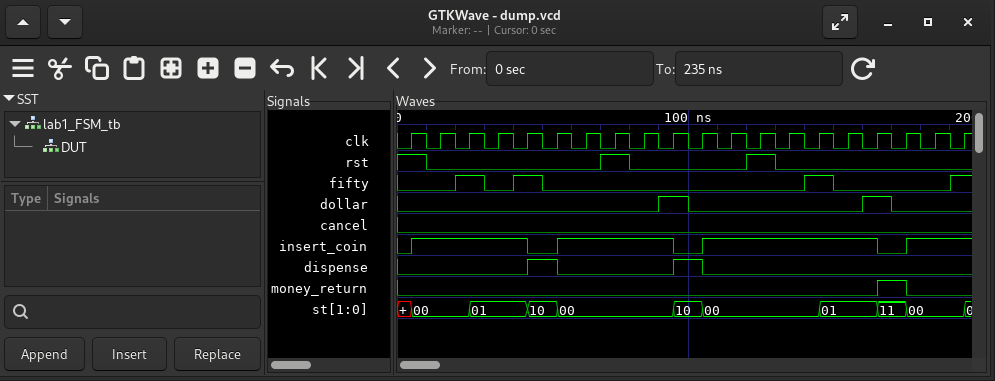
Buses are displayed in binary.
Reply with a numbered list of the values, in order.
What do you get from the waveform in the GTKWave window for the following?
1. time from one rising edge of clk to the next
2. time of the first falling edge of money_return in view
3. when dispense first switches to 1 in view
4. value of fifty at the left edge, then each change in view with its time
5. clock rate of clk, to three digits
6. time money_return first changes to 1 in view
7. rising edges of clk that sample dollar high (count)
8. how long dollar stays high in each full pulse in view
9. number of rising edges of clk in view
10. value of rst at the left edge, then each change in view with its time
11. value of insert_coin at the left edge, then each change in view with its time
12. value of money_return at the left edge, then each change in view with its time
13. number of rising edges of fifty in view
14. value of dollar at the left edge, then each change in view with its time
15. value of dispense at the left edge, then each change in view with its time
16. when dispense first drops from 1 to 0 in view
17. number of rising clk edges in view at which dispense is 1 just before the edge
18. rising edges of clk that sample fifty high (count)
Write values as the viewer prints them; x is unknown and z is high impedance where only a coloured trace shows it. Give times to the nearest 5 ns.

1. 10 ns
2. 175 ns
3. 45 ns
4. 0, 1 at 20 ns, 0 at 30 ns, 1 at 40 ns, 0 at 50 ns, 1 at 140 ns, 0 at 150 ns, 1 at 190 ns
5. 100 MHz
6. 165 ns
7. 2
8. 10 ns, 10 ns
9. 20
10. 1, 0 at 10 ns, 1 at 70 ns, 0 at 80 ns, 1 at 120 ns, 0 at 130 ns
11. 0, 1 at 5 ns, 0 at 45 ns, 1 at 55 ns, 0 at 95 ns, 1 at 105 ns, 0 at 165 ns, 1 at 175 ns
12. 0, 1 at 165 ns, 0 at 175 ns
13. 4
14. 0, 1 at 90 ns, 0 at 100 ns, 1 at 160 ns, 0 at 170 ns
15. 0, 1 at 45 ns, 0 at 55 ns, 1 at 95 ns, 0 at 105 ns
16. 55 ns
17. 2
18. 4
